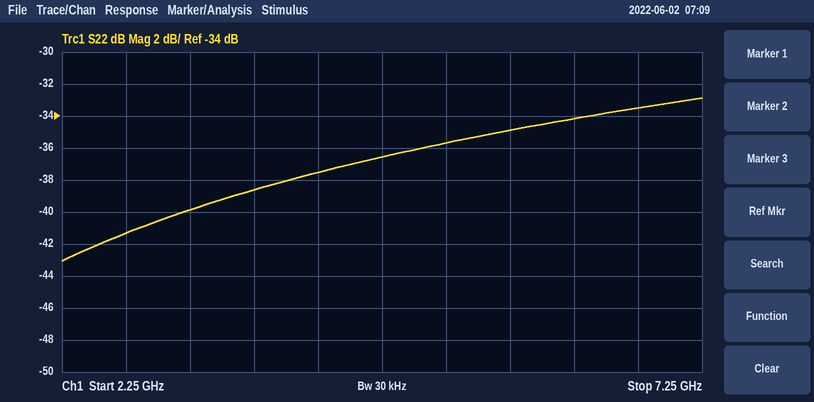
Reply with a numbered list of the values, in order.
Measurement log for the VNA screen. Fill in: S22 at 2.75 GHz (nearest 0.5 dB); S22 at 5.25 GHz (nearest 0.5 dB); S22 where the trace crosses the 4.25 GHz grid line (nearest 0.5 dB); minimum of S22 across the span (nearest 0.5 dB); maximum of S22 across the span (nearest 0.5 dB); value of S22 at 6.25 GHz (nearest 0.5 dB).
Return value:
1. -41.5 dB
2. -35.5 dB
3. -37.5 dB
4. -43.0 dB
5. -33.0 dB
6. -34.0 dB
